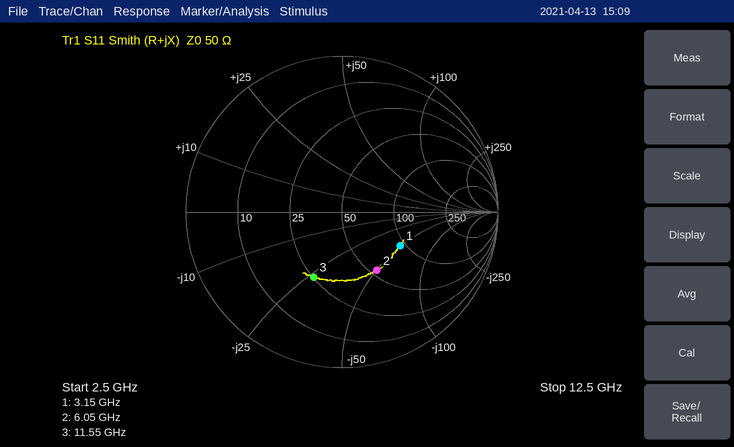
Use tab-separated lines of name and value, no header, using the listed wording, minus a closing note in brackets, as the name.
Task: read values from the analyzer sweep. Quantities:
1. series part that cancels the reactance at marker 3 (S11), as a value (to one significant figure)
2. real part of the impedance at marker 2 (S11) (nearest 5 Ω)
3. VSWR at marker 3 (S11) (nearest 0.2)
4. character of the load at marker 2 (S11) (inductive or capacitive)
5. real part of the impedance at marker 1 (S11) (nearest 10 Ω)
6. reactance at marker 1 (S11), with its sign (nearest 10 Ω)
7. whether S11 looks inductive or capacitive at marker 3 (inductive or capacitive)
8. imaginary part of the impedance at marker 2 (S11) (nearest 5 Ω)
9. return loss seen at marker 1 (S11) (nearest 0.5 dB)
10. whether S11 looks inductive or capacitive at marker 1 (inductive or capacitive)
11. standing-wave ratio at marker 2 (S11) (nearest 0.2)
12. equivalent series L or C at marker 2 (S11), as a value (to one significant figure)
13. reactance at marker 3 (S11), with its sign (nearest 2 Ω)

series part that cancels the reactance at marker 3 (S11), as a value	400 pH
real part of the impedance at marker 2 (S11)	55 Ω
VSWR at marker 3 (S11)	2.6
character of the load at marker 2 (S11)	capacitive
real part of the impedance at marker 1 (S11)	90 Ω
reactance at marker 1 (S11), with its sign	-50 Ω
whether S11 looks inductive or capacitive at marker 3	capacitive
imaginary part of the impedance at marker 2 (S11)	-50 Ω
return loss seen at marker 1 (S11)	7.5 dB
whether S11 looks inductive or capacitive at marker 1	capacitive
standing-wave ratio at marker 2 (S11)	2.6
equivalent series L or C at marker 2 (S11), as a value	500 fF
reactance at marker 3 (S11), with its sign	-26 Ω
